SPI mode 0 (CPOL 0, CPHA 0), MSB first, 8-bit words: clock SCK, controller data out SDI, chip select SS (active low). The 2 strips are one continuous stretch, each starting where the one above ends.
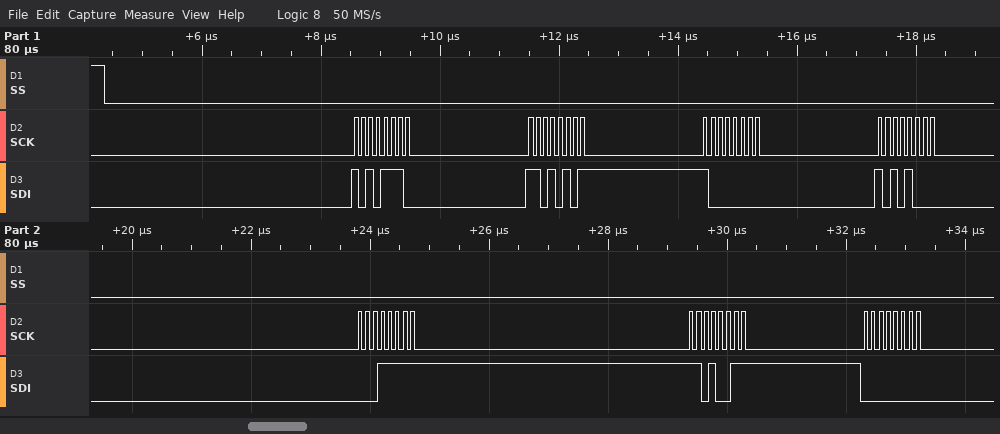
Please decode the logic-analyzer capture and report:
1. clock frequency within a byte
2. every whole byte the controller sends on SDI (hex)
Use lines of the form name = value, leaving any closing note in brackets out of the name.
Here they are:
clock frequency within a byte = 8 MHz
every whole byte the controller sends on SDI = 0xAE 0xD5 0x80 0xA8 0x1F 0xD3 0x00
